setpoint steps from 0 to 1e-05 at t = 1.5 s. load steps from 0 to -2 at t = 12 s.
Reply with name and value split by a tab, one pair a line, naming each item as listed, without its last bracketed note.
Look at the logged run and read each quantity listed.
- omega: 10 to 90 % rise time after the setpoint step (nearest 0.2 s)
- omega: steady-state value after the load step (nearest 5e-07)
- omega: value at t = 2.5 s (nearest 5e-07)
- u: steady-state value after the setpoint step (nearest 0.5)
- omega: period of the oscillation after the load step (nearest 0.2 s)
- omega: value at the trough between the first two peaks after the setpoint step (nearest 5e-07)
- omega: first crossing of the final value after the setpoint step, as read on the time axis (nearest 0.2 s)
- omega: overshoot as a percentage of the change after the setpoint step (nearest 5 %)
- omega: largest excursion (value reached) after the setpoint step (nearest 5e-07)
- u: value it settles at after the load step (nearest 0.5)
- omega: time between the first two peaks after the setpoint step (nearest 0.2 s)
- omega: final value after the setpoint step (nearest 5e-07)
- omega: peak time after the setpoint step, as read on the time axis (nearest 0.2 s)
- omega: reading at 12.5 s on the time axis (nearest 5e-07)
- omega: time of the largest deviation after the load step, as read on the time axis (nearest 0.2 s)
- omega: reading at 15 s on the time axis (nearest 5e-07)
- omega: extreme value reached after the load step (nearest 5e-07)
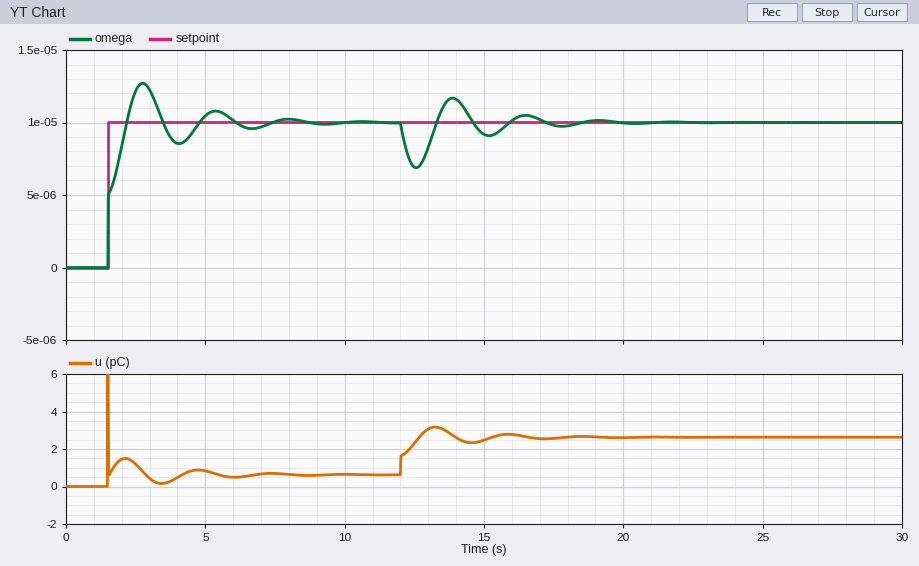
omega: 10 to 90 % rise time after the setpoint step	0.6 s
omega: steady-state value after the load step	0.0000100
omega: value at t = 2.5 s	0.0000120
u: steady-state value after the setpoint step	0.5
omega: period of the oscillation after the load step	2.6 s
omega: value at the trough between the first two peaks after the setpoint step	0.0000085
omega: first crossing of the final value after the setpoint step, as read on the time axis	2.2 s
omega: overshoot as a percentage of the change after the setpoint step	25 %
omega: largest excursion (value reached) after the setpoint step	0.0000125
u: value it settles at after the load step	2.5
omega: time between the first two peaks after the setpoint step	2.6 s
omega: final value after the setpoint step	0.0000100
omega: peak time after the setpoint step, as read on the time axis	2.8 s
omega: reading at 12.5 s on the time axis	0.0000070
omega: time of the largest deviation after the load step, as read on the time axis	12.6 s
omega: reading at 15 s on the time axis	0.0000090
omega: extreme value reached after the load step	0.0000070
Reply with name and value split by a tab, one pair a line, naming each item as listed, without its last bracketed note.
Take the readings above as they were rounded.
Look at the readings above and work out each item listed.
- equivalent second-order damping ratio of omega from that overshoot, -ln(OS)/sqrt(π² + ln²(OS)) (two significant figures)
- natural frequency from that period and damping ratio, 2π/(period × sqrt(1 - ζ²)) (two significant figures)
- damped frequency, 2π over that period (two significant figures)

equivalent second-order damping ratio of omega from that overshoot, -ln(OS)/sqrt(π² + ln²(OS))	0.40
natural frequency from that period and damping ratio, 2π/(period × sqrt(1 - ζ²))	2.6 rad/s
damped frequency, 2π over that period	2.4 rad/s
